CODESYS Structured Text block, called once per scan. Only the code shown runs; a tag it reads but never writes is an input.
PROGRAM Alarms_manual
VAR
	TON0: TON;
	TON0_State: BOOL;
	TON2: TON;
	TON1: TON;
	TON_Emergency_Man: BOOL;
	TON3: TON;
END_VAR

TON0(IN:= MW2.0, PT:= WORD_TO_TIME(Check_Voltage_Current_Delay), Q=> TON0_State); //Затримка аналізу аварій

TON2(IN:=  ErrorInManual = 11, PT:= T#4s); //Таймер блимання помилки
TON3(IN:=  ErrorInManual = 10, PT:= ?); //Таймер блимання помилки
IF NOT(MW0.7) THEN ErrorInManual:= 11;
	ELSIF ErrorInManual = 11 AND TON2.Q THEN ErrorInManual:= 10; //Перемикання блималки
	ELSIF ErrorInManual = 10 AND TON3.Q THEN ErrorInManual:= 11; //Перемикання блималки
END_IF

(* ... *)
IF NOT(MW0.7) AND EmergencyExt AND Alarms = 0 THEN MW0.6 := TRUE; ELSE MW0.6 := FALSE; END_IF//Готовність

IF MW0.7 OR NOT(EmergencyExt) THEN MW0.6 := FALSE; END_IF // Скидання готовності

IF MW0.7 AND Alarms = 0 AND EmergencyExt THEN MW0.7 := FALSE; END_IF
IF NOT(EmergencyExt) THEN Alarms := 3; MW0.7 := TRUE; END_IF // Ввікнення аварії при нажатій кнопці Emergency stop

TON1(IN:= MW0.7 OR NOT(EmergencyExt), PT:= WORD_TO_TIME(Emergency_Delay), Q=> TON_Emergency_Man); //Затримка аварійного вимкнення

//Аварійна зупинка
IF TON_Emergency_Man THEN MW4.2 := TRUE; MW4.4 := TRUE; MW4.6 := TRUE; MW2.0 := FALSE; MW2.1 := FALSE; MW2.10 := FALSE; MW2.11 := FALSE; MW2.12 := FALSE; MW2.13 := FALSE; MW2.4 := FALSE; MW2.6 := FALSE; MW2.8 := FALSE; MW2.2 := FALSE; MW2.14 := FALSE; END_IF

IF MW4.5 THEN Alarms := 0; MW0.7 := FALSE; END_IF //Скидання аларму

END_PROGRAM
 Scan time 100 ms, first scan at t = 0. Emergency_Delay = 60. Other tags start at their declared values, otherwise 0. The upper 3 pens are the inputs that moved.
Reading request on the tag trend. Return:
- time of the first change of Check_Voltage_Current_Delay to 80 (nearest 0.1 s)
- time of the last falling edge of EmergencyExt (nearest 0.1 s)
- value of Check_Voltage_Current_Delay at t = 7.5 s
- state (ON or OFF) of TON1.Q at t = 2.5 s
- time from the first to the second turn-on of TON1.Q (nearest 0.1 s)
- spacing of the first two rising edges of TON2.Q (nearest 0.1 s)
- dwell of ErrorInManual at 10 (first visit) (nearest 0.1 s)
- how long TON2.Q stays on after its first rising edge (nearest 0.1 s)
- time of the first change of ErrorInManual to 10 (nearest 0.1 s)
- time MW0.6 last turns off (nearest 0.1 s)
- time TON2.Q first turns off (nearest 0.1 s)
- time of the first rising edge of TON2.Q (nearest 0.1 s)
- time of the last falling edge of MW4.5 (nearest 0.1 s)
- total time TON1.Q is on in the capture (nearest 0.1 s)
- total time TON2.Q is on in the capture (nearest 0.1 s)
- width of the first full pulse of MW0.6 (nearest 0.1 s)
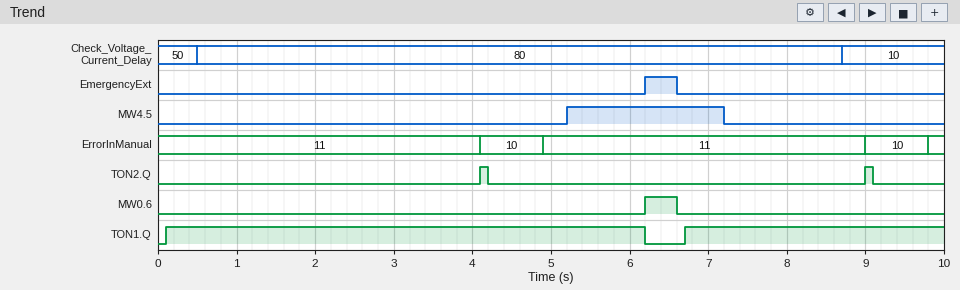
0.5 s
6.6 s
80
ON
6.6 s
4.9 s
0.8 s
0.1 s
4.1 s
6.6 s
4.2 s
4.1 s
7.2 s
9.4 s
0.2 s
0.4 s
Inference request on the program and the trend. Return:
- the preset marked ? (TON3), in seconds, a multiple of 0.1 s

0.7 s
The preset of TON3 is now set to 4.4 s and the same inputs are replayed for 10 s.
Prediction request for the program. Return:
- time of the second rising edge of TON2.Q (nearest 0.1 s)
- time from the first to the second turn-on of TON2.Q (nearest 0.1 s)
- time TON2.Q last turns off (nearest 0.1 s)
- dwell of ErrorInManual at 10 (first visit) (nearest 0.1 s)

9.4 s
5.3 s
9.5 s
1.2 s
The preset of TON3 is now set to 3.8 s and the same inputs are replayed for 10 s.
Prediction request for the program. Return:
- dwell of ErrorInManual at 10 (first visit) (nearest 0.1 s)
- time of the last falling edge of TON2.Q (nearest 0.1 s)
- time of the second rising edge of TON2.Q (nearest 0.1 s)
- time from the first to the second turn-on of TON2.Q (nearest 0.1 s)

1.2 s
9.5 s
9.4 s
5.3 s
